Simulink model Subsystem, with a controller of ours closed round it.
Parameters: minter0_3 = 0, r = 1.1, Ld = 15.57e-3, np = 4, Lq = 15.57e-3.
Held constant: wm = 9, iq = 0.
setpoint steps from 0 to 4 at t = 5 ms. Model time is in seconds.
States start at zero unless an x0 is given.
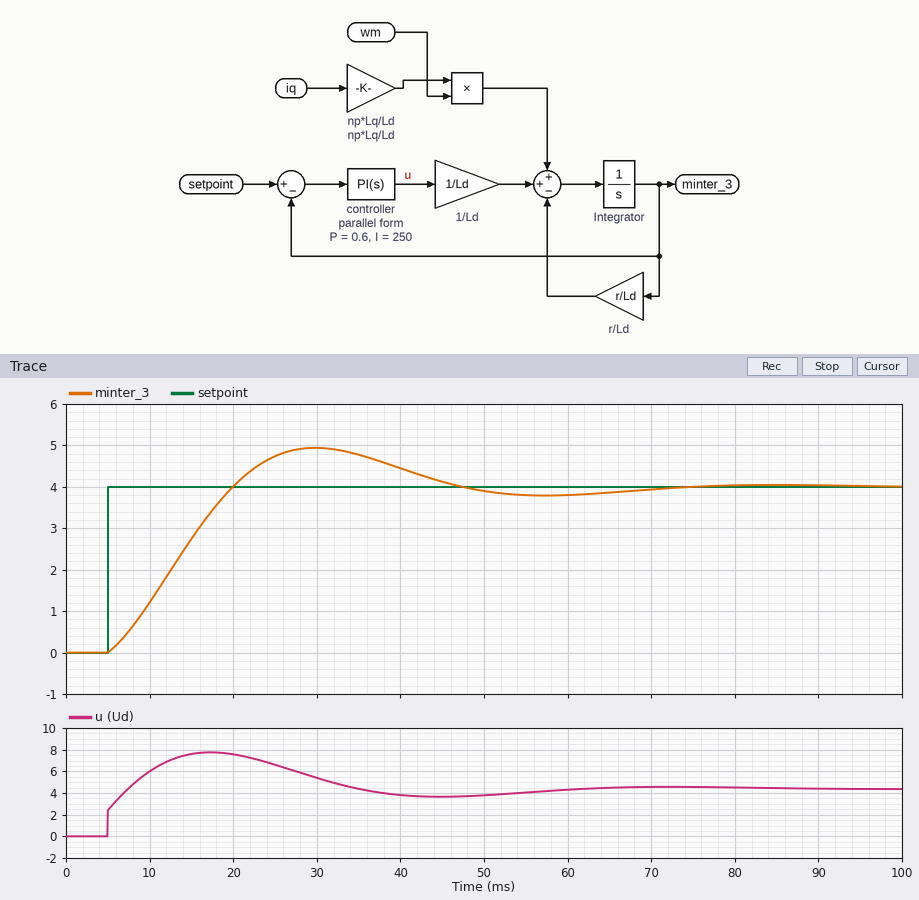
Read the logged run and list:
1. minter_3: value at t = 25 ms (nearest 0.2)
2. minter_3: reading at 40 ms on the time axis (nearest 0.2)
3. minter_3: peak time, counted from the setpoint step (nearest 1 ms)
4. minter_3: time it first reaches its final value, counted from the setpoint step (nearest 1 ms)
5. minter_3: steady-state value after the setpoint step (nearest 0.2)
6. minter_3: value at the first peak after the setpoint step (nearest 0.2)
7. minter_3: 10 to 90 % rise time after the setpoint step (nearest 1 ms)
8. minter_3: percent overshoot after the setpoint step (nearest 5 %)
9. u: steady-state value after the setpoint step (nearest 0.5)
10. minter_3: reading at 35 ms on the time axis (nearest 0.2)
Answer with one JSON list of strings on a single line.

["4.8", "4.4", "25 ms", "15 ms", "4.0", "5.0", "11 ms", "25 %", "4.5", "4.8"]
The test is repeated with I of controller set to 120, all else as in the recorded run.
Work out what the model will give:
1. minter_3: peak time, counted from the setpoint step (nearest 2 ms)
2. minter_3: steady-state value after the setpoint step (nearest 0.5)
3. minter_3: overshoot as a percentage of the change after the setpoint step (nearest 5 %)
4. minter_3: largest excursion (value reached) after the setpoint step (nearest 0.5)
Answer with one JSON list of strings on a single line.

["40 ms", "4.0", "10 %", "4.5"]
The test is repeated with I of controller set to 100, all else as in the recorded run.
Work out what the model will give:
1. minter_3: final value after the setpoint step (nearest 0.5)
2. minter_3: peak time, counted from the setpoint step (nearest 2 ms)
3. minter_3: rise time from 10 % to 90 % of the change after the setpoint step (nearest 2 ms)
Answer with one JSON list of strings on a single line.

["4.0", "46 ms", "22 ms"]
